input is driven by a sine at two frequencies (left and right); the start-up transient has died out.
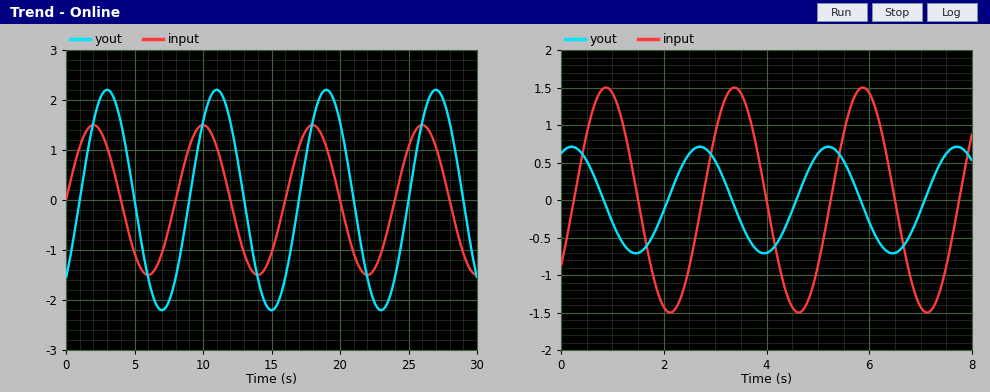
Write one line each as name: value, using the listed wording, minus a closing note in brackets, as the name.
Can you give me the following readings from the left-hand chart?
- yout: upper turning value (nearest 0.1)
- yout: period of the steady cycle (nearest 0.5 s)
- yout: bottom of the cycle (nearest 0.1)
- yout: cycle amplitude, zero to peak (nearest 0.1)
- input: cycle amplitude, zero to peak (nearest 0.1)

yout: upper turning value: 2.2
yout: period of the steady cycle: 8.0 s
yout: bottom of the cycle: -2.2
yout: cycle amplitude, zero to peak: 2.2
input: cycle amplitude, zero to peak: 1.5
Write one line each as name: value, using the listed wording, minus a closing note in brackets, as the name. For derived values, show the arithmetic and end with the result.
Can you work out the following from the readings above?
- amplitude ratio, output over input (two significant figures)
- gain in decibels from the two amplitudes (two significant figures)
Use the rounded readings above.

amplitude ratio, output over input: 2.2 / 1.5 = 1.5
gain in decibels from the two amplitudes: 20 log10(2.2 / 1.5) = 3.3 dB
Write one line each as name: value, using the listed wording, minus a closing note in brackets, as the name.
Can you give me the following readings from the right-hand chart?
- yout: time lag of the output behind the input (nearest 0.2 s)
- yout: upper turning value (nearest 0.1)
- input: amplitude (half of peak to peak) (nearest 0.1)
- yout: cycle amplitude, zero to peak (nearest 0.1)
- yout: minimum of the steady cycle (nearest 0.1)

yout: time lag of the output behind the input: 1.8 s
yout: upper turning value: 0.7
input: amplitude (half of peak to peak): 1.5
yout: cycle amplitude, zero to peak: 0.7
yout: minimum of the steady cycle: -0.7
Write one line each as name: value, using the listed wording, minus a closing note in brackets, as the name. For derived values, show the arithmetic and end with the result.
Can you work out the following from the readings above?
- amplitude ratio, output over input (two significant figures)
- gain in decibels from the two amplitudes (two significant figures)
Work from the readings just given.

amplitude ratio, output over input: 0.7 / 1.5 = 0.47
gain in decibels from the two amplitudes: 20 log10(0.7 / 1.5) = -6.6 dB
